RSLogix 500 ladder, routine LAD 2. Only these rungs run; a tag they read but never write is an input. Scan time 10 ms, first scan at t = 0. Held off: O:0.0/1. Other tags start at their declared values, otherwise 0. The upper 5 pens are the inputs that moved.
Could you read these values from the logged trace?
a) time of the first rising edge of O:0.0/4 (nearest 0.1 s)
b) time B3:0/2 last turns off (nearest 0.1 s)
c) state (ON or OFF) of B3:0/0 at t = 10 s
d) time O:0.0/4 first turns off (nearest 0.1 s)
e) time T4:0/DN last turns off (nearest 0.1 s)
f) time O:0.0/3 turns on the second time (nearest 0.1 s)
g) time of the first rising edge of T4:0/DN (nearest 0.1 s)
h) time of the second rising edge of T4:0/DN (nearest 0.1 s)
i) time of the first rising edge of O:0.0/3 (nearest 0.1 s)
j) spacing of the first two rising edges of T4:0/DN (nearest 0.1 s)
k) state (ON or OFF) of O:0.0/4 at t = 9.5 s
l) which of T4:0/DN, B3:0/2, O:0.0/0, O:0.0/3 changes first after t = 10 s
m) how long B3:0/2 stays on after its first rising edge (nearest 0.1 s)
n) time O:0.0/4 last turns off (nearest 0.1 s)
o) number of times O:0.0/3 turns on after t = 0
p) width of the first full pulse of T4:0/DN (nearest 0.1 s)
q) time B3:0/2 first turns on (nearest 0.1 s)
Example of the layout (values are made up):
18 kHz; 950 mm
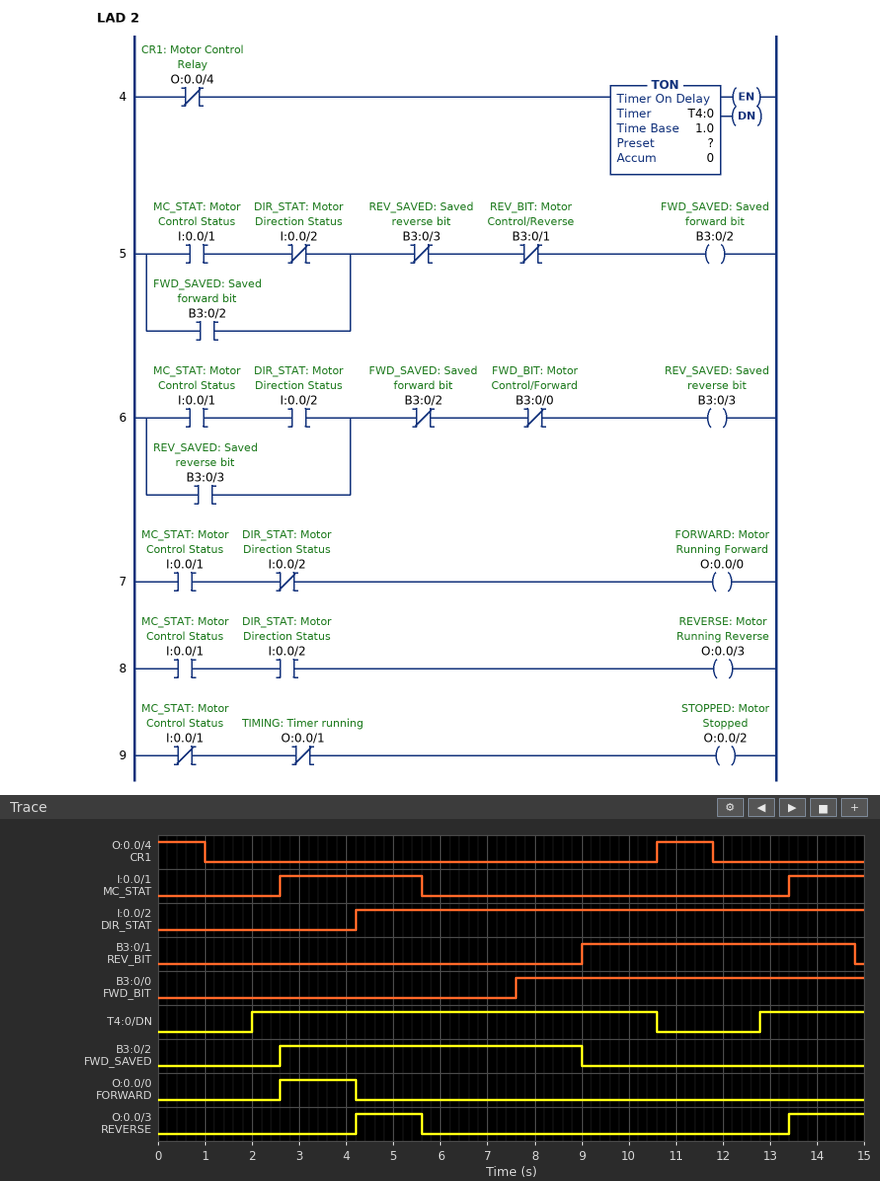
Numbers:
10.6 s; 9.0 s; ON; 1.0 s; 10.6 s; 13.4 s; 2.0 s; 12.8 s; 4.2 s; 10.8 s; OFF; T4:0/DN; 6.4 s; 11.8 s; 2; 8.6 s; 2.6 s
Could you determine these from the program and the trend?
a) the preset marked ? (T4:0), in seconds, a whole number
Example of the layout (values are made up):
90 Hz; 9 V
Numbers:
1 s
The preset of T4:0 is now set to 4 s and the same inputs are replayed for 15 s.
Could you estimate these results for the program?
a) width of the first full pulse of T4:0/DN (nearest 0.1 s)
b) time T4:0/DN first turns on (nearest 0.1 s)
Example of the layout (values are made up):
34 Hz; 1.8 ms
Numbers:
5.6 s; 5.0 s
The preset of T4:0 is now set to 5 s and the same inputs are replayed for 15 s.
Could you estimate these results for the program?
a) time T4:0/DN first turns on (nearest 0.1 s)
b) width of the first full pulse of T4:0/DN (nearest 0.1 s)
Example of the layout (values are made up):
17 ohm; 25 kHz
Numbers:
6.0 s; 4.6 s
